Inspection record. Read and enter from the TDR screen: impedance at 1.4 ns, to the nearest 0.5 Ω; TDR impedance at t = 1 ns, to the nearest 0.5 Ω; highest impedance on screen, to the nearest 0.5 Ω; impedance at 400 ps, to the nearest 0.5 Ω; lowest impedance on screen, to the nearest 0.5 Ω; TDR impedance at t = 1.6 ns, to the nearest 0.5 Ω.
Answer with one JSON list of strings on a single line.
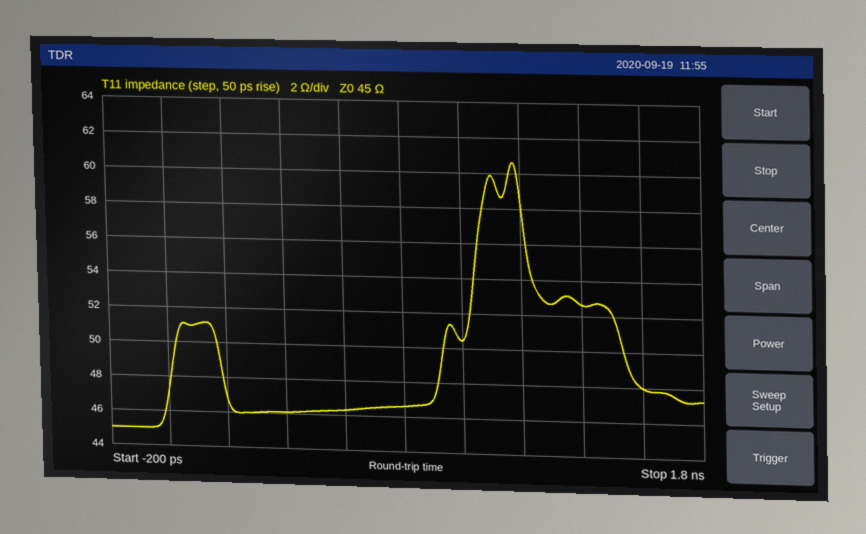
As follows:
["52.5 Ω", "50.5 Ω", "60.5 Ω", "46.0 Ω", "45.0 Ω", "48.0 Ω"]
